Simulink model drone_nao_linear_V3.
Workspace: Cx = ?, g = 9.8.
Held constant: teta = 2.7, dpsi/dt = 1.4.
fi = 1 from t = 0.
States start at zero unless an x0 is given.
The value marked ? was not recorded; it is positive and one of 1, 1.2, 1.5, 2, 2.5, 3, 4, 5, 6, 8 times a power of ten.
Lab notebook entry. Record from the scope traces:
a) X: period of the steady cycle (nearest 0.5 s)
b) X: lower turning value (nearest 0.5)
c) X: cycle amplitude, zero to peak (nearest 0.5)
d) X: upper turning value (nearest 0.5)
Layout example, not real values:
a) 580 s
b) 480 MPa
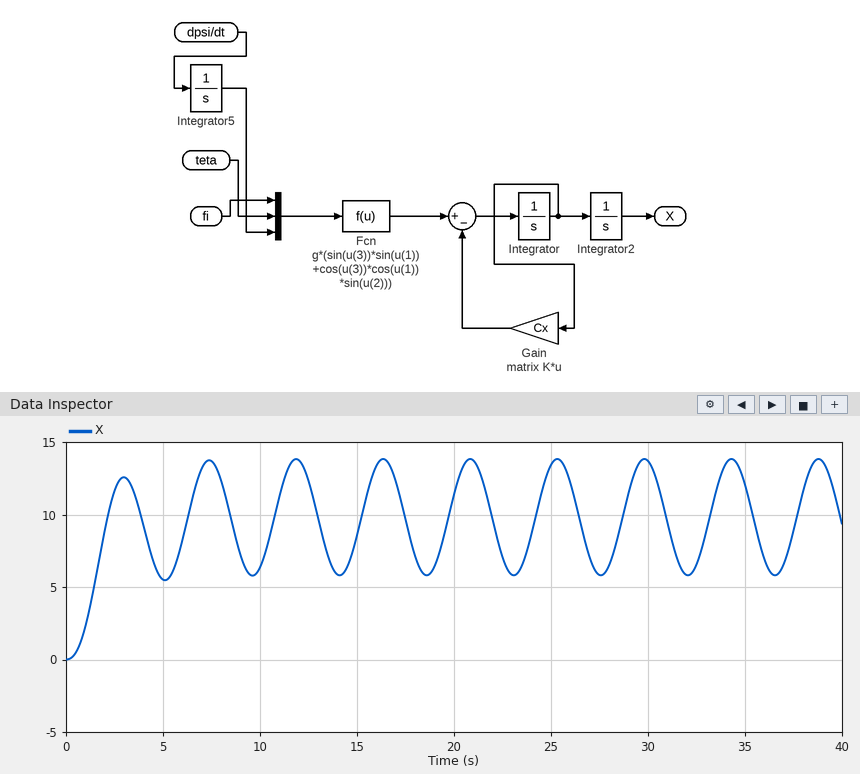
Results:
a) 4.5 s
b) 6.0
c) 4.0
d) 14.0
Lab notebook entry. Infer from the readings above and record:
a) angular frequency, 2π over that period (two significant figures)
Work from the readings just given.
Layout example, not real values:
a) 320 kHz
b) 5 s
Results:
a) 1.4 rad/s
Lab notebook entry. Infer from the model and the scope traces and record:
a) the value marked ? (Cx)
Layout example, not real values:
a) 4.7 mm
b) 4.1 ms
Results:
a) 0.6
